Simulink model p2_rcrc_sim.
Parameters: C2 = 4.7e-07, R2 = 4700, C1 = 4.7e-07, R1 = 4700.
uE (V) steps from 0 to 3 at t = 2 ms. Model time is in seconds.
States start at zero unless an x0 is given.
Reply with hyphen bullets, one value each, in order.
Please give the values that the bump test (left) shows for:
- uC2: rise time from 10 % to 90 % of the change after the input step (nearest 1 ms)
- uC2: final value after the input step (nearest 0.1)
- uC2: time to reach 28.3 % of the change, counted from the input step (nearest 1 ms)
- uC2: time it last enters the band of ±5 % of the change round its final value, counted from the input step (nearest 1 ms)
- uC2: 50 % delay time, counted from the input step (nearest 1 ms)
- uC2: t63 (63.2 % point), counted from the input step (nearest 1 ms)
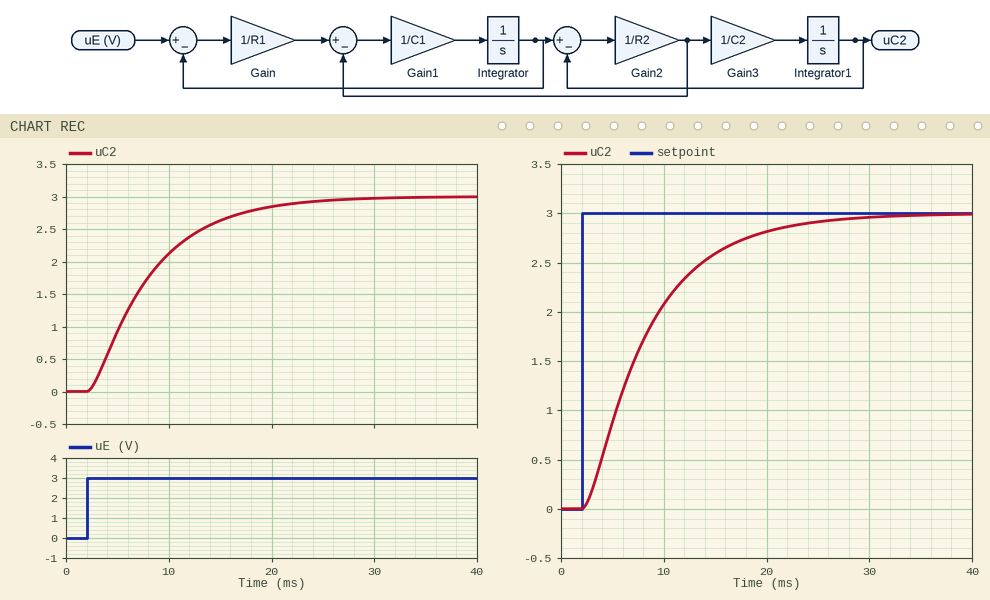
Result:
- 13 ms
- 3.0
- 3 ms
- 18 ms
- 5 ms
- 7 ms
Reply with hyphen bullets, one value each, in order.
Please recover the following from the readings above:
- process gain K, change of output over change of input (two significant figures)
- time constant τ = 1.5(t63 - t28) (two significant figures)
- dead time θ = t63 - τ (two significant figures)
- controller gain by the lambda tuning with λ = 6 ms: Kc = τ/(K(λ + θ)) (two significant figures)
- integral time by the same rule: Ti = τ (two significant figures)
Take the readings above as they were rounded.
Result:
- 1.0
- 6.0 ms
- 1.0 ms
- 0.86
- 6.0 ms
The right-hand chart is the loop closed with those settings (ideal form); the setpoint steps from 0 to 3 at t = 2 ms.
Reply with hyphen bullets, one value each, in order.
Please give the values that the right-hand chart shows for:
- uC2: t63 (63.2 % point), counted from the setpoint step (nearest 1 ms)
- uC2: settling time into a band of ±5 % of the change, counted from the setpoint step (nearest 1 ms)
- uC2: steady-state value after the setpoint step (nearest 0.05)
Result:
- 7 ms
- 19 ms
- 3.00
